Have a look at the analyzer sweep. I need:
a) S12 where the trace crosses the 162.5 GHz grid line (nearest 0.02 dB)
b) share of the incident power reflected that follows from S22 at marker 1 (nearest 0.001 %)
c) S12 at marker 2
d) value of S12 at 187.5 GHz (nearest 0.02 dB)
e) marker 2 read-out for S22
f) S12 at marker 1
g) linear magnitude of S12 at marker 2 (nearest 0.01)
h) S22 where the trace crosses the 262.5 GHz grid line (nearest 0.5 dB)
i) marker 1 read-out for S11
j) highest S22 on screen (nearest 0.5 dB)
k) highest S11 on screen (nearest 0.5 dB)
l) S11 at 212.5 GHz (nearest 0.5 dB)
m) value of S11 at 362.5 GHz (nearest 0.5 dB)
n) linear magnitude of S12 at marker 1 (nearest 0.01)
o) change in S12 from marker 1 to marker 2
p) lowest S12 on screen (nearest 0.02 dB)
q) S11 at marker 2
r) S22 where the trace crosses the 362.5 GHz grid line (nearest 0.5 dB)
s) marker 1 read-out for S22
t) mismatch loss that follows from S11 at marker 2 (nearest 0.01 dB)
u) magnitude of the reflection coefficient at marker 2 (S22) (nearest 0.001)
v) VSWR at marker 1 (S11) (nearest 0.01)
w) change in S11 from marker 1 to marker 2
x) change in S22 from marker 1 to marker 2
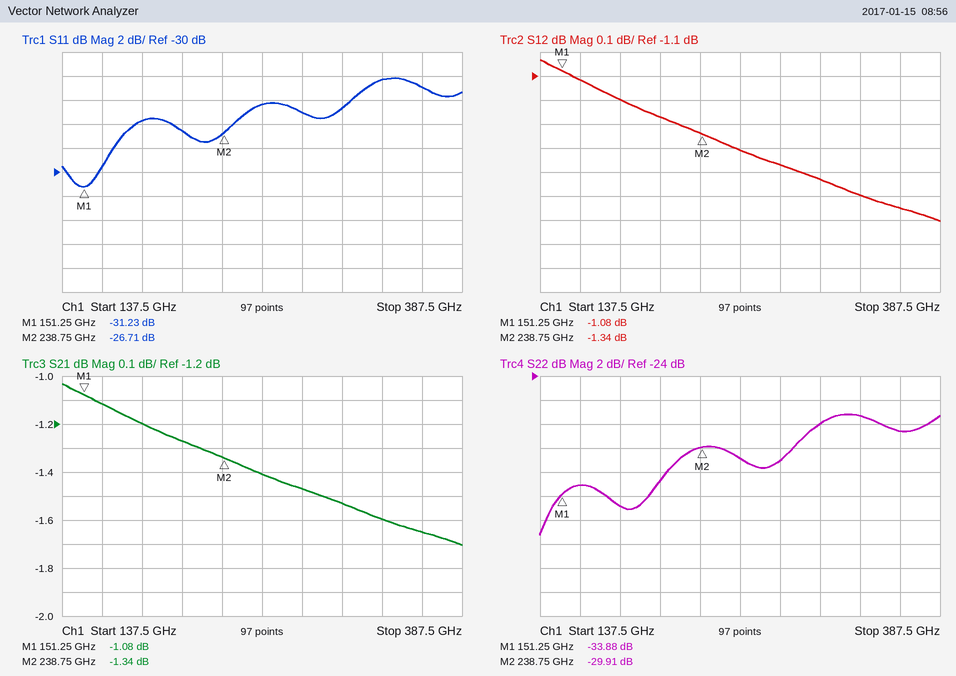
-1.12 dB
0.041 %
-1.34 dB
-1.20 dB
-29.91 dB
-1.08 dB
0.86
-31.0 dB
-31.23 dB
-27.0 dB
-22.0 dB
-26.5 dB
-23.0 dB
0.88
-0.26 dB
-1.70 dB
-26.71 dB
-28.5 dB
-33.88 dB
0.01 dB
0.032
1.06
4.52 dB
3.97 dB
